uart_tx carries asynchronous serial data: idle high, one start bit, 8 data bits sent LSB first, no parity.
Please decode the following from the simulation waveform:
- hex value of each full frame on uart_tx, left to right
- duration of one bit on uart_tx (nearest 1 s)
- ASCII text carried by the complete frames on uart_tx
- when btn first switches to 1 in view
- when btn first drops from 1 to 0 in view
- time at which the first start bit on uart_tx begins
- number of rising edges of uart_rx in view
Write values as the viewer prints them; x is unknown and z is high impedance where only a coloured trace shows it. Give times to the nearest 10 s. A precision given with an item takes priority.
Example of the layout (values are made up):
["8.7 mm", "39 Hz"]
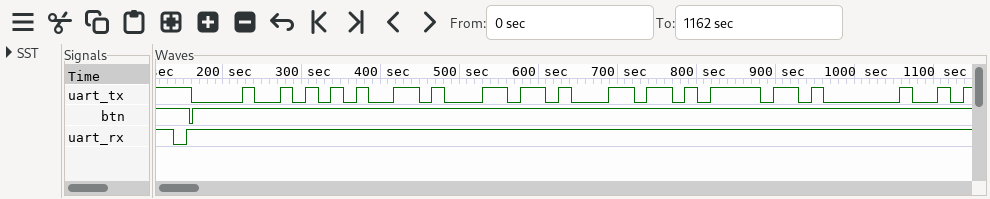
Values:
["48, 65, 6C, 6C, 6F, 20", "16 s", "\"Hello \"", "160 s", "160 s", "160 s", "1"]
